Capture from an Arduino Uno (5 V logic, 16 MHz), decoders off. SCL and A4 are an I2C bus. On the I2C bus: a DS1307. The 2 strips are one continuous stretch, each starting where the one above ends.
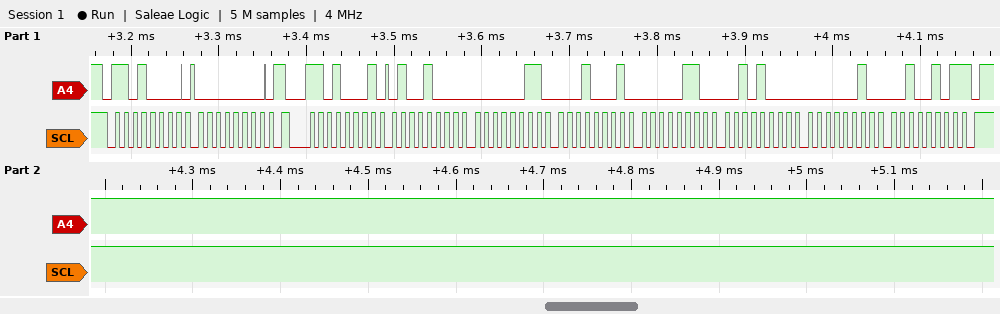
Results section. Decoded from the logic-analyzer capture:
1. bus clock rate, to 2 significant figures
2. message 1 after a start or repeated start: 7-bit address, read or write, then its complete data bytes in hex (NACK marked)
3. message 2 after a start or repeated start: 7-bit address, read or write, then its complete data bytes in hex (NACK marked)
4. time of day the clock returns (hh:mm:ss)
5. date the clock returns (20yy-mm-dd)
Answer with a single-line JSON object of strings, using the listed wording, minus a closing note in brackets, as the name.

{"bus clock rate, to 2 significant figures": "100 kHz", "message 1 after a start or repeated start: 7-bit address, read or write, then its complete data bytes in hex": "0x68 write: 00", "message 2 after a start or repeated start: 7-bit address, read or write, then its complete data bytes in hex": "0x68 read: 48 03 11 06 28 02 25 NACK", "time of day the clock returns": "11:03:48", "date the clock returns": "2025-02-28"}
